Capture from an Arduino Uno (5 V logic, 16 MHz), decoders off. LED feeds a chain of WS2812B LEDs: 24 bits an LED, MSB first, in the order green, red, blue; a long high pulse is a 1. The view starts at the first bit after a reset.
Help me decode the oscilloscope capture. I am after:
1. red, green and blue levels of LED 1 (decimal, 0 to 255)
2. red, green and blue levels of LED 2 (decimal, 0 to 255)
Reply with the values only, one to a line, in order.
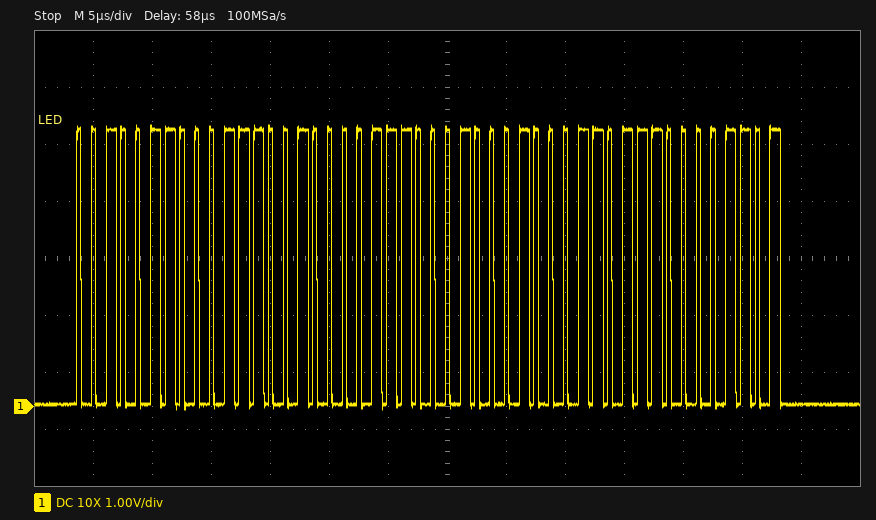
57, 38, 14
55, 34, 13
